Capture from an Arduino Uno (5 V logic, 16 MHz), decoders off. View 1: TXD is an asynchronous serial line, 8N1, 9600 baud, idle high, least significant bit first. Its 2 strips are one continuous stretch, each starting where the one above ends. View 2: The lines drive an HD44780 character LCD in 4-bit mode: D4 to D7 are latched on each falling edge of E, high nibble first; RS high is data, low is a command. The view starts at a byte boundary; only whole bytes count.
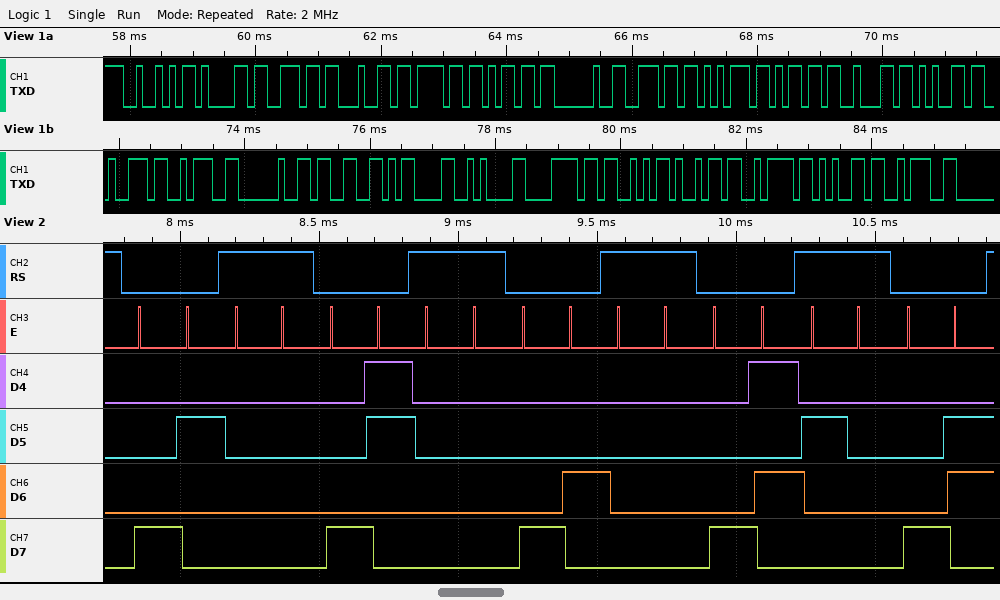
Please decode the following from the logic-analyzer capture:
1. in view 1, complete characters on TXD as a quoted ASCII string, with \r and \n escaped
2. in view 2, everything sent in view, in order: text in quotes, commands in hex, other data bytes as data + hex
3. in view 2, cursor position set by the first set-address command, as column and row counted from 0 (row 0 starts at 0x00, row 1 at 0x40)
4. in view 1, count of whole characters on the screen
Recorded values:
"Random number: 3\r\nxSize:"
0x82 data 00 0x83 data 00 0x84 data 00 0x85 " " 0x86
column 2, row 0
24
